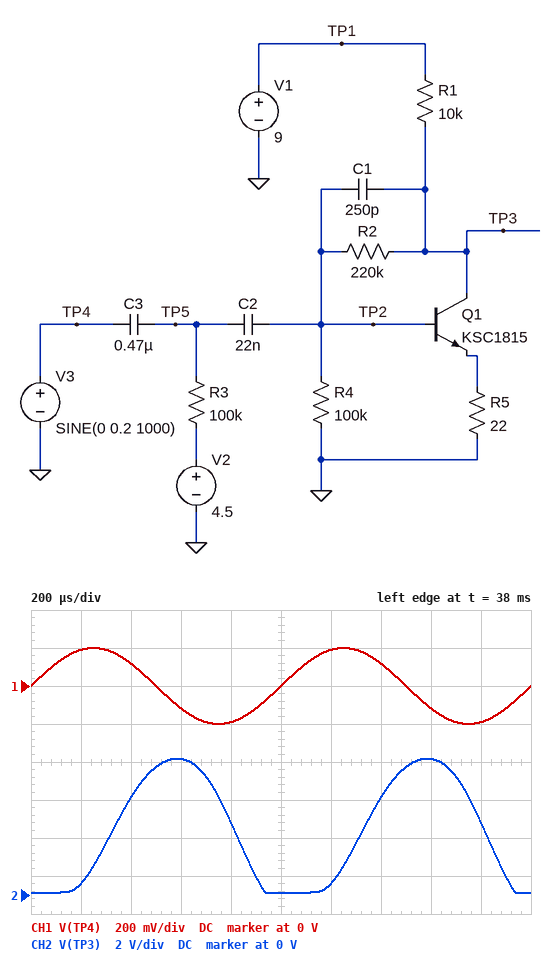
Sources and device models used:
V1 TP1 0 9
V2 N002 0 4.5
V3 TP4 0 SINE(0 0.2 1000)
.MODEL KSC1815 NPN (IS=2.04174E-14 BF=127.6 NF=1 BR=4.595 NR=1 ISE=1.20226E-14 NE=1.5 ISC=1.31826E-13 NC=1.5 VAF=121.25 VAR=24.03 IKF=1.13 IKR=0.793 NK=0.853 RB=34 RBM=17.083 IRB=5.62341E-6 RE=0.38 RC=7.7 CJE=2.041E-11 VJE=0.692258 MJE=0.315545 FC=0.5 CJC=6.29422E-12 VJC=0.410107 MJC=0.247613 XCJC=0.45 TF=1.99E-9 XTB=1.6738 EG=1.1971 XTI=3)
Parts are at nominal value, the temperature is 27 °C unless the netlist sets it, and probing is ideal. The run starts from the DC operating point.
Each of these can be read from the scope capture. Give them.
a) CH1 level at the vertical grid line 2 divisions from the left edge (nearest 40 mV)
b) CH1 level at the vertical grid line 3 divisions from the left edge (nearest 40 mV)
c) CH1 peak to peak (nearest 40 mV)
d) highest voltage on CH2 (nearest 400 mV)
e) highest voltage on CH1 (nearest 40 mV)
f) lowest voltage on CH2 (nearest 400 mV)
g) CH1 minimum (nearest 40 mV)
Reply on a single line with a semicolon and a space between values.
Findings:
120 mV; -120 mV; 400 mV; 7.2 V; 200 mV; 0 V; -200 mV
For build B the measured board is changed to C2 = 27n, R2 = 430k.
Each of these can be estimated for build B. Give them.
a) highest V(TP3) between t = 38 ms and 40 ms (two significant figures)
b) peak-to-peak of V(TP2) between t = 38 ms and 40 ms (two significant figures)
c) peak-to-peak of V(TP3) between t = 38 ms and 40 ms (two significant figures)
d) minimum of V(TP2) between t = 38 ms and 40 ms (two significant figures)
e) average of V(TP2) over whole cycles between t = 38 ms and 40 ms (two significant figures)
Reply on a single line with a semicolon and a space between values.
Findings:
8.8 V; 190 mV; 8.7 V; 470 mV; 580 mV
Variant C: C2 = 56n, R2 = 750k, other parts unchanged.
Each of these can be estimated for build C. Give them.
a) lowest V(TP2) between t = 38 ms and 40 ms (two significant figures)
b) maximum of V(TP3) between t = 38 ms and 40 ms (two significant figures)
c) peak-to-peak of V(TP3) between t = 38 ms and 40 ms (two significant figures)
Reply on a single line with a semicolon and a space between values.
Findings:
320 mV; 8.9 V; 8.8 V
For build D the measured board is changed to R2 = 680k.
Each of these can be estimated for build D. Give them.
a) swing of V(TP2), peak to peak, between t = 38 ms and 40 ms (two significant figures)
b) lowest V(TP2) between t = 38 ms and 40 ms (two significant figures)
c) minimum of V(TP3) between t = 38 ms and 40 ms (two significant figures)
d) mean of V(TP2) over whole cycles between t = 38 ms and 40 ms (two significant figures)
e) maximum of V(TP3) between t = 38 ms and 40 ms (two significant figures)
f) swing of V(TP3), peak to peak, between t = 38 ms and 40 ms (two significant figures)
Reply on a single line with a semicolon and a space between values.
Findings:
240 mV; 410 mV; 150 mV; 550 mV; 8.9 V; 8.7 V
